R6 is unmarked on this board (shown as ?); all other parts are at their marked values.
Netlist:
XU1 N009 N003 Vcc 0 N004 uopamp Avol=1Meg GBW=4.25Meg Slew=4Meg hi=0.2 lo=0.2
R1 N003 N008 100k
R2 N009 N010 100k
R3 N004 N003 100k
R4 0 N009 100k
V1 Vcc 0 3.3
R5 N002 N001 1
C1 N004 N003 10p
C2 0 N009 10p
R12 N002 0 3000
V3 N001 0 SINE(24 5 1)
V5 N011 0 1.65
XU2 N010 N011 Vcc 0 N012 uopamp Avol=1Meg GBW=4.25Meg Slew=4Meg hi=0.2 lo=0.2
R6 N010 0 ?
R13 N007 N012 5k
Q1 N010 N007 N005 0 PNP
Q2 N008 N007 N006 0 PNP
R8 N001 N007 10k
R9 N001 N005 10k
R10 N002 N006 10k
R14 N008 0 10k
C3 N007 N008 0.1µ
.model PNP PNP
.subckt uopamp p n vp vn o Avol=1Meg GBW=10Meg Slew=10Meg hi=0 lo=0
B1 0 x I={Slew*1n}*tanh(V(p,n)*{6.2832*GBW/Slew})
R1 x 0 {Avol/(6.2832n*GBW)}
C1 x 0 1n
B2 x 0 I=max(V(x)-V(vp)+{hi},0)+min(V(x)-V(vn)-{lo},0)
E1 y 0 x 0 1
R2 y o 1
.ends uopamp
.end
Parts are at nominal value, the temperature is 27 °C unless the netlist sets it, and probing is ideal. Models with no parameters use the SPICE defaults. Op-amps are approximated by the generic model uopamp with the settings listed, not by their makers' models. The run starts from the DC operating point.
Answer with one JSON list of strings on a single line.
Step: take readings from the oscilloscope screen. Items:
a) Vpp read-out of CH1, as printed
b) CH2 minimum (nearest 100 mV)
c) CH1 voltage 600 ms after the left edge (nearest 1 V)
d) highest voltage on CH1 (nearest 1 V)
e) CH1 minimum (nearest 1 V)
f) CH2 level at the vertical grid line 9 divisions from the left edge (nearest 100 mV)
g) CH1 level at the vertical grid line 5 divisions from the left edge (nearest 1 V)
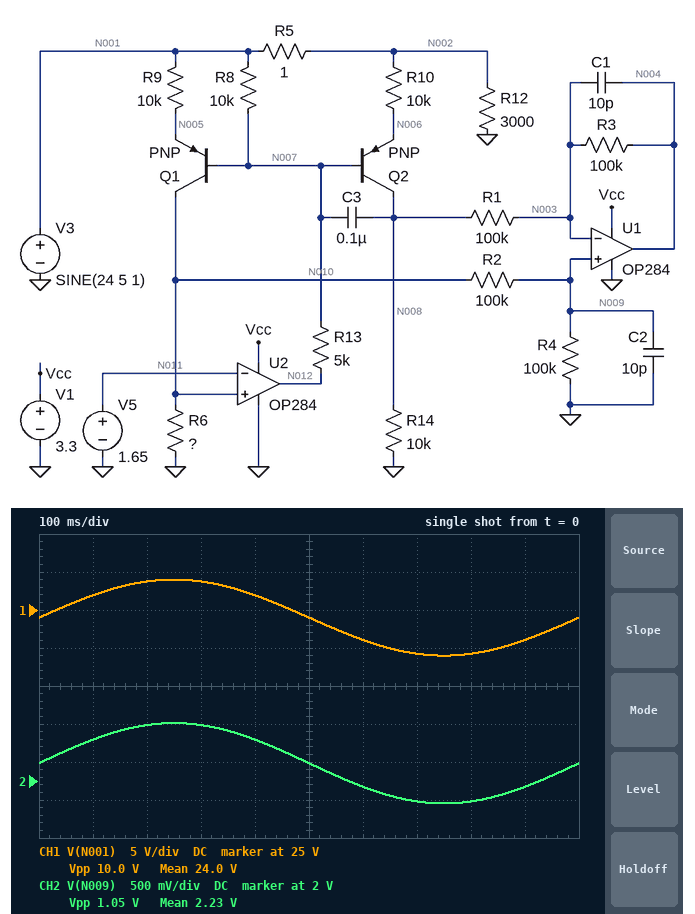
["10.0 V", "1.7 V", "21 V", "29 V", "19 V", "1.9 V", "24 V"]
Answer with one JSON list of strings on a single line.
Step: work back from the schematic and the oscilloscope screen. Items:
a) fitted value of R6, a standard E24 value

["3.6 kΩ"]
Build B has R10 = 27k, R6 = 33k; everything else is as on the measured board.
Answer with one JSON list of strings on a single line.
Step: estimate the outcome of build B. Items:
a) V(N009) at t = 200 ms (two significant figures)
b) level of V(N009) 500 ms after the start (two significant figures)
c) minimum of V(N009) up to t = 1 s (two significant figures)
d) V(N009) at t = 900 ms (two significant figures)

["7.6 V", "6.5 V", "5.3 V", "5.8 V"]
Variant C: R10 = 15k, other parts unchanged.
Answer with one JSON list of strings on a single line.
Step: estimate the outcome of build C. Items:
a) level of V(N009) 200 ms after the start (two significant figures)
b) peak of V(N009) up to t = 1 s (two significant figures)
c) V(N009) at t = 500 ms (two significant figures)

["2.8 V", "2.9 V", "2.3 V"]
